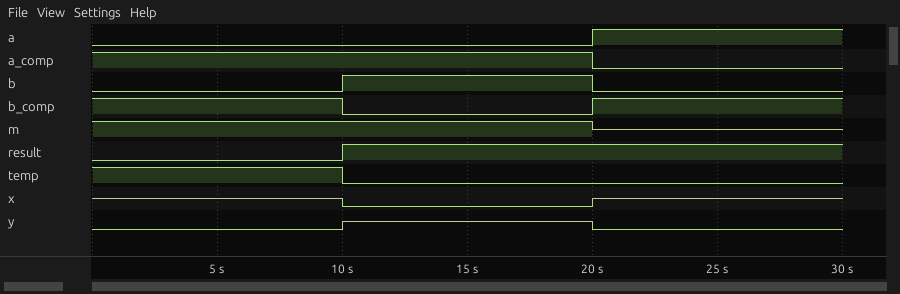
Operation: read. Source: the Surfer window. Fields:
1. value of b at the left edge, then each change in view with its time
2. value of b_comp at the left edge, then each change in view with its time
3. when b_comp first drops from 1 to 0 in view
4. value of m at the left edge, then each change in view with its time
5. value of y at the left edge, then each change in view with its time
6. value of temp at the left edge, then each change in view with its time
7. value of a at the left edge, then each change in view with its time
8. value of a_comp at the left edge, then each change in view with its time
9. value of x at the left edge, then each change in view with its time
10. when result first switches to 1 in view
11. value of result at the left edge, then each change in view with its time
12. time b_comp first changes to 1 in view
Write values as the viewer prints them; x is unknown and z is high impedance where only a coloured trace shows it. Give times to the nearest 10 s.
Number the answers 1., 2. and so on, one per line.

1. 0, 1 at 10 s, 0 at 20 s
2. 1, 0 at 10 s, 1 at 20 s
3. 10 s
4. 1, z at 20 s
5. 0, z at 10 s, 0 at 20 s
6. 1, 0 at 10 s
7. 0, 1 at 20 s
8. 1, 0 at 20 s
9. z, 0 at 10 s, z at 20 s
10. 10 s
11. 0, 1 at 10 s
12. 20 s
